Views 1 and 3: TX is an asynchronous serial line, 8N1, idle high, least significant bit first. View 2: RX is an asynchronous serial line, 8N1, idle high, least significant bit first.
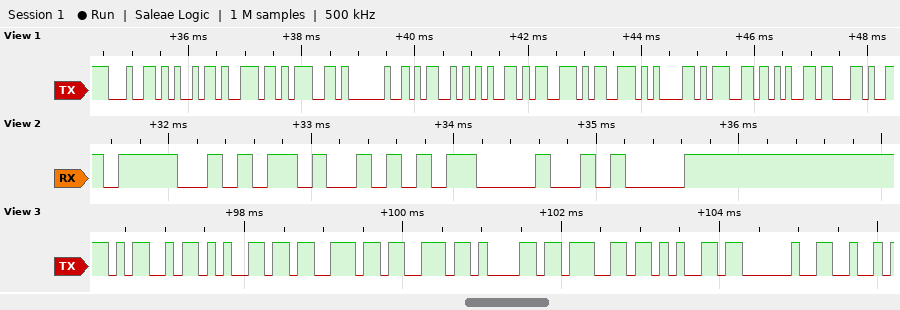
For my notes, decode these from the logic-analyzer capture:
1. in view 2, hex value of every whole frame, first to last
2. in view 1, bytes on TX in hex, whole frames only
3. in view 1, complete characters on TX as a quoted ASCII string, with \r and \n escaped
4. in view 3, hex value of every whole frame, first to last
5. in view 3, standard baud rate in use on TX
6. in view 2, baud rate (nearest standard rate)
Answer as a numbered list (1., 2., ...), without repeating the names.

1. 4F 4B 0D 0A
2. 64 69 6E 67 20 4D 65 73 73 61 67 65 2C
3. "ding Message,"
4. 4D 65 73 73 61 67 65 20
5. 9600 baud
6. 9600 baud
